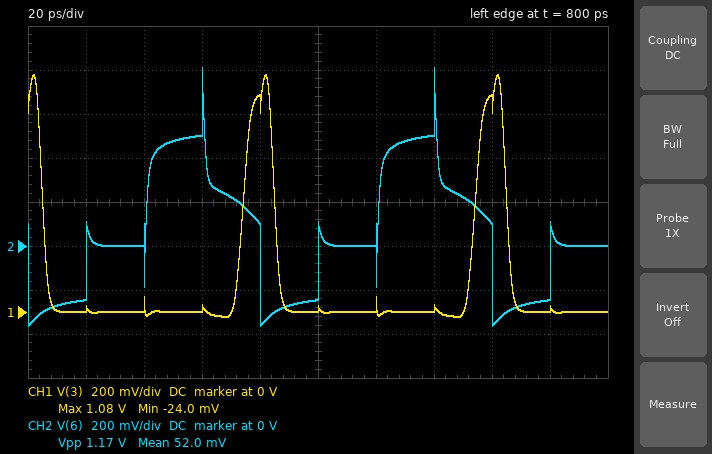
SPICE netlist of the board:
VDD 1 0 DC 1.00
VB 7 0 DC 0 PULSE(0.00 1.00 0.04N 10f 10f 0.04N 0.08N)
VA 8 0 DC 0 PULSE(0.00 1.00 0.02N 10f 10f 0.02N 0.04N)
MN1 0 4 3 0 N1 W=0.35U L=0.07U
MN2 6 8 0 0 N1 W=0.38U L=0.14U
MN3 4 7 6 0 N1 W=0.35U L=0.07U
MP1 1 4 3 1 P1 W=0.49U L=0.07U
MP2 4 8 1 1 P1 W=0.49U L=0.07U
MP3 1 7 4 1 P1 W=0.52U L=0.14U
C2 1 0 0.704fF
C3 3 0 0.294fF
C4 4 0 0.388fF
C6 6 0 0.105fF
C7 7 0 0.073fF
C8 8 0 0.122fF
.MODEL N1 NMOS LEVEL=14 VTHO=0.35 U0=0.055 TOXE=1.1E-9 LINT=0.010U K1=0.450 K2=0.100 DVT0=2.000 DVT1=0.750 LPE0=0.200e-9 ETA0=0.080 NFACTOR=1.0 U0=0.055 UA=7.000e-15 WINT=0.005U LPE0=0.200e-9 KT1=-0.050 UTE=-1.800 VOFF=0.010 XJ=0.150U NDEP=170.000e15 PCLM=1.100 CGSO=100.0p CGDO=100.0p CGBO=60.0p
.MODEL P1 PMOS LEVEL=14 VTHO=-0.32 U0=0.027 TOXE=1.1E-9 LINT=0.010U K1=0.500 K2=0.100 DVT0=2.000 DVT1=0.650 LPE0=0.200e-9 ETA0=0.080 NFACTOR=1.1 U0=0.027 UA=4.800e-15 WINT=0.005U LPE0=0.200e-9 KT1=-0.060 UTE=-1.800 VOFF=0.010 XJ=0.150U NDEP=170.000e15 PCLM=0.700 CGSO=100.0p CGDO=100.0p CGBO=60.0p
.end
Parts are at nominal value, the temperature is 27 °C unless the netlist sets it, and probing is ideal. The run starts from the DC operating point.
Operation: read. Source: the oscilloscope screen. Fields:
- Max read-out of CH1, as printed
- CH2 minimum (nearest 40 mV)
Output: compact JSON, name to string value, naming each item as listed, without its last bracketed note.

{"Max read-out of CH1, as printed": "1.08 V", "CH2 minimum": "-360 mV"}
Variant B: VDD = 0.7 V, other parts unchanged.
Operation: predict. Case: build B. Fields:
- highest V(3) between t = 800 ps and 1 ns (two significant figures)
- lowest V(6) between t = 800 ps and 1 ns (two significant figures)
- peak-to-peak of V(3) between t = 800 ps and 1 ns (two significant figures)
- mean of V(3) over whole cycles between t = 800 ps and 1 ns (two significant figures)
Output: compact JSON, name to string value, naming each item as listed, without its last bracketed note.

{"highest V(3) between t = 800 ps and 1 ns": "800 mV", "lowest V(6) between t = 800 ps and 1 ns": "-420 mV", "peak-to-peak of V(3) between t = 800 ps and 1 ns": "870 mV", "mean of V(3) over whole cycles between t = 800 ps and 1 ns": "120 mV"}
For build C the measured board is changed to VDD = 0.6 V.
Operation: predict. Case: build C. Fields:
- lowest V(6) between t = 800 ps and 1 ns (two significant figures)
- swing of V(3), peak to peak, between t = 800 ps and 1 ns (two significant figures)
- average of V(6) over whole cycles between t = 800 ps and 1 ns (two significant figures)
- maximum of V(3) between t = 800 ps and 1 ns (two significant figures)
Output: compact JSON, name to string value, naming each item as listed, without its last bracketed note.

{"lowest V(6) between t = 800 ps and 1 ns": "-440 mV", "swing of V(3), peak to peak, between t = 800 ps and 1 ns": "780 mV", "average of V(6) over whole cycles between t = 800 ps and 1 ns": "62 mV", "maximum of V(3) between t = 800 ps and 1 ns": "690 mV"}
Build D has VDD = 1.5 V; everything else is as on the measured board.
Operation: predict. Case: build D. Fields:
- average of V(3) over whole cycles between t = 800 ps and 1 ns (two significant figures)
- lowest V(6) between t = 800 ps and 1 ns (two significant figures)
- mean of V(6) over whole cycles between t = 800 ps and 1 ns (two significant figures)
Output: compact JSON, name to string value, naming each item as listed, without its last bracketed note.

{"average of V(3) over whole cycles between t = 800 ps and 1 ns": "57 mV", "lowest V(6) between t = 800 ps and 1 ns": "-210 mV", "mean of V(6) over whole cycles between t = 800 ps and 1 ns": "150 mV"}
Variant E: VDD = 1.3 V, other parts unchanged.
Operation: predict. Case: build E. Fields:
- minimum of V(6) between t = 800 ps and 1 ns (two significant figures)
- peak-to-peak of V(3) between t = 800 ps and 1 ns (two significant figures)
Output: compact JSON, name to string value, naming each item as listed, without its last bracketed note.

{"minimum of V(6) between t = 800 ps and 1 ns": "-280 mV", "peak-to-peak of V(3) between t = 800 ps and 1 ns": "1.4 V"}
